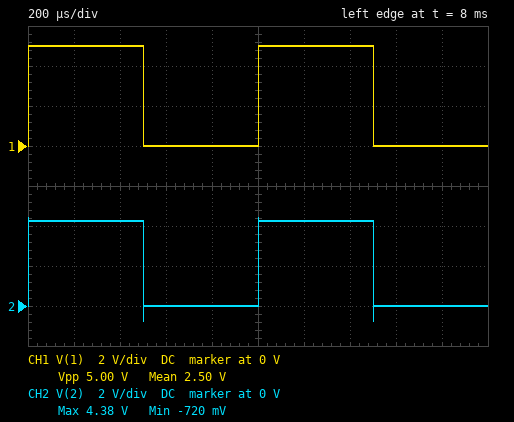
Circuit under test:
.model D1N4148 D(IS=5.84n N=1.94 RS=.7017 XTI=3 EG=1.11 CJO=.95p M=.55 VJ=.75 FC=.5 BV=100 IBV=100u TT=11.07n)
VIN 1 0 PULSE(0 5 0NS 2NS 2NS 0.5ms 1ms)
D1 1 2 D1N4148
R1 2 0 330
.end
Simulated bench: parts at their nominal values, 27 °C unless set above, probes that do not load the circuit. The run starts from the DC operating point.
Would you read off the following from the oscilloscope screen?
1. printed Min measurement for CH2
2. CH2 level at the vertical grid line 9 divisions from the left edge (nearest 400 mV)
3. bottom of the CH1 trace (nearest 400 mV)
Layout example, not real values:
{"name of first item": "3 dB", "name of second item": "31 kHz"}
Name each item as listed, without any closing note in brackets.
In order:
{"printed Min measurement for CH2": "-720 mV", "CH2 level at the vertical grid line 9 divisions from the left edge": "0 V", "bottom of the CH1 trace": "0 V"}
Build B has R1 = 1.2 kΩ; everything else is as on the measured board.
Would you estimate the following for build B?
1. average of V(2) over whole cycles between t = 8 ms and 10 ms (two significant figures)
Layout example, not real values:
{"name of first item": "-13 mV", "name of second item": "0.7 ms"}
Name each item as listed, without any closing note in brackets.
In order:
{"average of V(2) over whole cycles between t = 8 ms and 10 ms": "2.2 V"}
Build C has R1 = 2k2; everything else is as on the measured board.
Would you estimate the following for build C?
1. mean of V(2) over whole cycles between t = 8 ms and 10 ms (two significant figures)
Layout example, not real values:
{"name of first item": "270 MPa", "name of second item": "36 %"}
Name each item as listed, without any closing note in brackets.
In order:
{"mean of V(2) over whole cycles between t = 8 ms and 10 ms": "2.2 V"}
